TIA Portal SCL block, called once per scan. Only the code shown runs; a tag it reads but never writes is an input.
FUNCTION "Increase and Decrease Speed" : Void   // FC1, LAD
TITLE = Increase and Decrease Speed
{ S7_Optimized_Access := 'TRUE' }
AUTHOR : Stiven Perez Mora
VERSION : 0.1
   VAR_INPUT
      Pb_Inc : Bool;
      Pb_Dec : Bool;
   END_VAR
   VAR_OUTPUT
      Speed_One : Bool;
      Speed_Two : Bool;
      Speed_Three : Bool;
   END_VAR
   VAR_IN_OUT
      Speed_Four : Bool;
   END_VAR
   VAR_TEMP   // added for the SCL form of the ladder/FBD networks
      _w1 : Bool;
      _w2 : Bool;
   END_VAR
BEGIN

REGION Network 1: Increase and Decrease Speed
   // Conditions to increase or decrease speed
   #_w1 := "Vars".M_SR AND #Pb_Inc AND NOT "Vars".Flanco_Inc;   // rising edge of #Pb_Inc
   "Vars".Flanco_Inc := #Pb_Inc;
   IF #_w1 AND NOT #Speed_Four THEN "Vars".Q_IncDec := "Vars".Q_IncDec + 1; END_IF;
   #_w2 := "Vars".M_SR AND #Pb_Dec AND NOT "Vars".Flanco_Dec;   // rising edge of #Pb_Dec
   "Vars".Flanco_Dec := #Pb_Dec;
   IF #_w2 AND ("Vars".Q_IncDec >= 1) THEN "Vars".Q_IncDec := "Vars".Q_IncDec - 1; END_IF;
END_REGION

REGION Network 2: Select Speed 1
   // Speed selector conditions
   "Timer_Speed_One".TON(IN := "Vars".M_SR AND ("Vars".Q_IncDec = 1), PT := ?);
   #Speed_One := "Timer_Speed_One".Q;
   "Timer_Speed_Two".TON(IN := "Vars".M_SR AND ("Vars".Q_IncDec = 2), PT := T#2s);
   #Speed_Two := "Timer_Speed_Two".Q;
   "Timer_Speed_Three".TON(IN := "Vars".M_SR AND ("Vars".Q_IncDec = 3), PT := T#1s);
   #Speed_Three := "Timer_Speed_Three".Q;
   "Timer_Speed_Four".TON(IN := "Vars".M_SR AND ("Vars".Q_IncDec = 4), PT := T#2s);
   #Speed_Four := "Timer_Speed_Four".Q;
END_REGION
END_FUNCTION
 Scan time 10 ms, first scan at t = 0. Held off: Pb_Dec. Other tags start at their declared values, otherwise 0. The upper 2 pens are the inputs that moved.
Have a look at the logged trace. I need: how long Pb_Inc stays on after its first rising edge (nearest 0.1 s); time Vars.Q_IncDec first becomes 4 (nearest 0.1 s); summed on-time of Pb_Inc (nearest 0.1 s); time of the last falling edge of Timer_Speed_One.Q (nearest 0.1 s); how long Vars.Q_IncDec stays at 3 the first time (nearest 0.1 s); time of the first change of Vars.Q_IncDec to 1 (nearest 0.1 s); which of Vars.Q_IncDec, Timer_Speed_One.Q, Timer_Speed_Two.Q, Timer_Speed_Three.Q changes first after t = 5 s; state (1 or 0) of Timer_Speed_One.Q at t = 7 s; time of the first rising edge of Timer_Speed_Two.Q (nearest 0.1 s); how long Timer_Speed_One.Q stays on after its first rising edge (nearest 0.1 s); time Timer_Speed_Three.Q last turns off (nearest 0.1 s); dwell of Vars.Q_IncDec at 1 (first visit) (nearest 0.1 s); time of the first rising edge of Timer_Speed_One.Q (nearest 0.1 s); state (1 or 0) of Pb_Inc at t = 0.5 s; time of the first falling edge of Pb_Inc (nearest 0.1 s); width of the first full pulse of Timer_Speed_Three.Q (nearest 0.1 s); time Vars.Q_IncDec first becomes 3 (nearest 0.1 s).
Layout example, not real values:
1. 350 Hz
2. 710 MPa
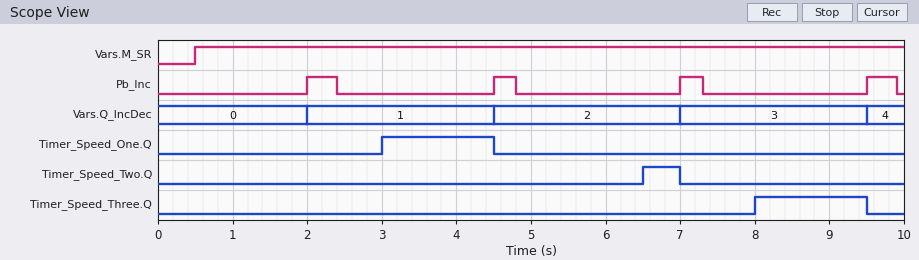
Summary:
1. 0.4 s
2. 9.5 s
3. 1.4 s
4. 4.5 s
5. 2.5 s
6. 2.0 s
7. Timer_Speed_Two.Q
8. 0
9. 6.5 s
10. 1.5 s
11. 9.5 s
12. 2.5 s
13. 3.0 s
14. 0
15. 2.4 s
16. 1.5 s
17. 7.0 s
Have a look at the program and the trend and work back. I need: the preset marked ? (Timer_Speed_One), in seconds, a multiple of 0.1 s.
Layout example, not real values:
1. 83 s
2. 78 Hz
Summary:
1. 1.0 s
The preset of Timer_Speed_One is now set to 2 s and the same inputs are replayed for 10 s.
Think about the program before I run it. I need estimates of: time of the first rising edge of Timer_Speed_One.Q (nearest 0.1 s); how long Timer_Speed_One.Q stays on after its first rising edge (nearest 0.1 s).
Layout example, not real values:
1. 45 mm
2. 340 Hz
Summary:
1. 4.0 s
2. 0.5 s
